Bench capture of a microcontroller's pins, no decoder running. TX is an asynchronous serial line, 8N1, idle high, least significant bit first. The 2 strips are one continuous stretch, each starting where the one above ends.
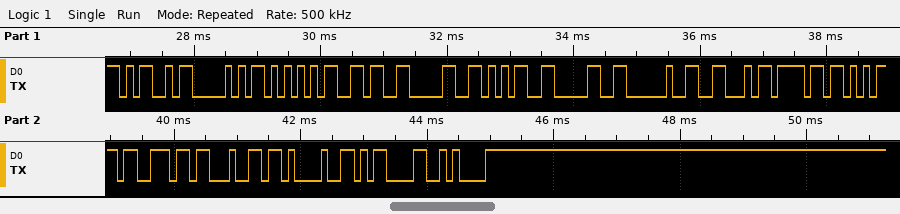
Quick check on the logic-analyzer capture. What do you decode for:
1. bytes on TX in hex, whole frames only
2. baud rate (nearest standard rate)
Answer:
4D 50 55 36 30 35 30 20 46 6F 75 6E 64 21 0D 0A
9600 baud
